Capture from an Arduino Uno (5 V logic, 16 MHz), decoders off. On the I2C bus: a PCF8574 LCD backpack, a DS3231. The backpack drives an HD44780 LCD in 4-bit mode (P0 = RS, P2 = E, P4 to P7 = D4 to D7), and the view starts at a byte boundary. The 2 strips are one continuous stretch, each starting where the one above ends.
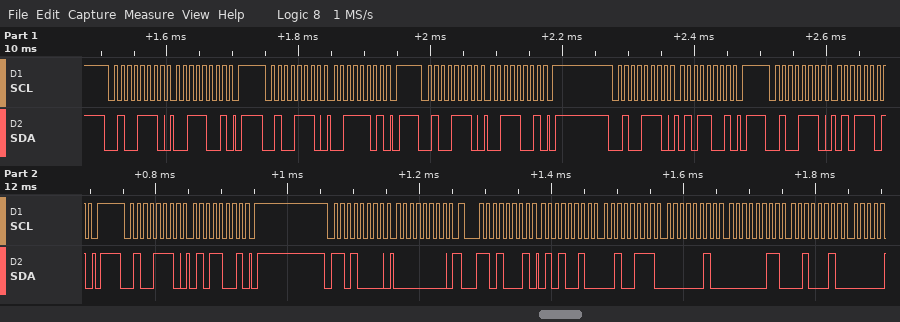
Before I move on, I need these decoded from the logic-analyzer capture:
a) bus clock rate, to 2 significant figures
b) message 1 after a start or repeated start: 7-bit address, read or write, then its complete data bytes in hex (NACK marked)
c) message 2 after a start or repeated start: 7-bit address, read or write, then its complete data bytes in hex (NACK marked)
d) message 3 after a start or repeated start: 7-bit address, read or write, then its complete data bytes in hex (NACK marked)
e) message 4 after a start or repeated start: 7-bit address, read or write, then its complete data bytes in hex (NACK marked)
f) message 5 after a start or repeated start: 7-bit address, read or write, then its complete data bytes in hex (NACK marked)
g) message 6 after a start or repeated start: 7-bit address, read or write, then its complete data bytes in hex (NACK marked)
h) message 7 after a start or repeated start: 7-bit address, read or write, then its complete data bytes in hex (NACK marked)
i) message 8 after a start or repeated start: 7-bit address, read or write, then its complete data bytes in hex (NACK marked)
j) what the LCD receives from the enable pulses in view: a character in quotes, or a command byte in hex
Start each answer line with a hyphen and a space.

- 100 kHz
- 0x27 write: 39
- 0x27 write: 3D
- 0x27 write: 39
- 0x27 write: 59
- 0x27 write: 5D
- 0x27 write: 59
- 0x68 write: 00
- 0x68 read: 52 27 02 03 22
- '5'
